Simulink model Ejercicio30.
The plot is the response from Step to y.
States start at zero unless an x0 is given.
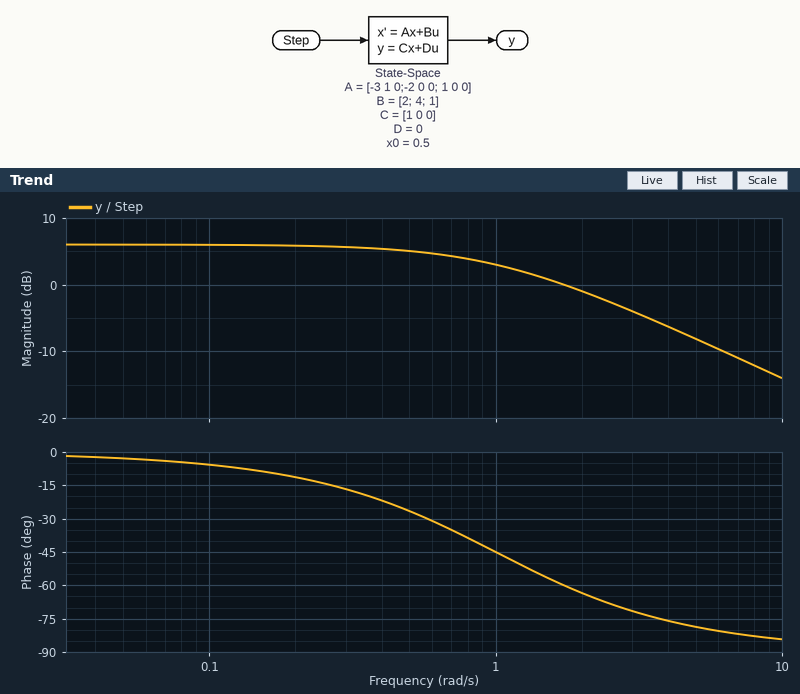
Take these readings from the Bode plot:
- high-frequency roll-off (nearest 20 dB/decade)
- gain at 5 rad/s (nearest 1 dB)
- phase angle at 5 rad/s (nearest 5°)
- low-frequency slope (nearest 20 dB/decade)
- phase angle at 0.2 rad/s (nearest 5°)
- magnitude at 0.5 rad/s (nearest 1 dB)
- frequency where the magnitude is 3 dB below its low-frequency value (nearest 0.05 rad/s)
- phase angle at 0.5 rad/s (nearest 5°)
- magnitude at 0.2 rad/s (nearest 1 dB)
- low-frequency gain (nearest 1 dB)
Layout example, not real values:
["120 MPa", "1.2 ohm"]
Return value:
["-20 dB/decade", "-8 dB", "-80°", "0 dB/decade", "-10°", "5 dB", "1.00 rad/s", "-25°", "6 dB", "6 dB"]
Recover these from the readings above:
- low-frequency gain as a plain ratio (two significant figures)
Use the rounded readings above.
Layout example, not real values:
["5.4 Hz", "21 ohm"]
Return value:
["2.0"]
